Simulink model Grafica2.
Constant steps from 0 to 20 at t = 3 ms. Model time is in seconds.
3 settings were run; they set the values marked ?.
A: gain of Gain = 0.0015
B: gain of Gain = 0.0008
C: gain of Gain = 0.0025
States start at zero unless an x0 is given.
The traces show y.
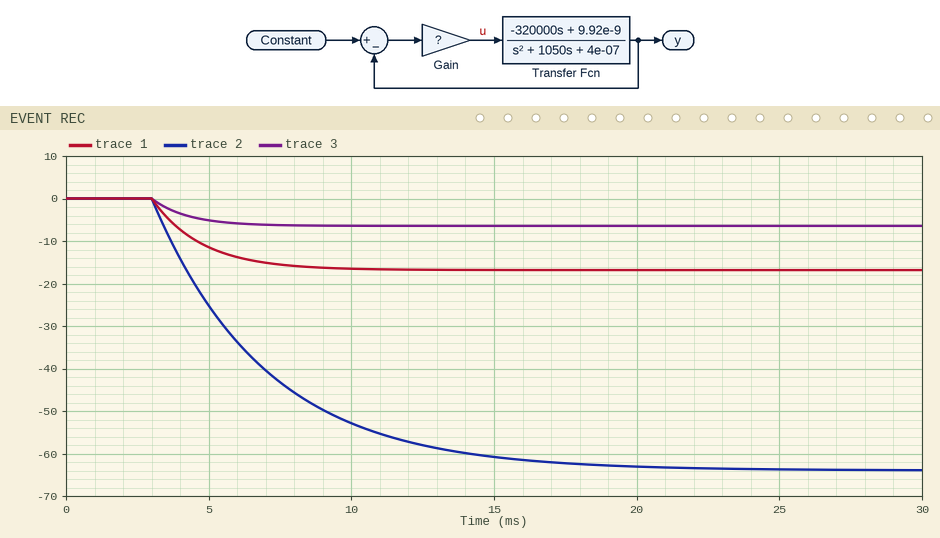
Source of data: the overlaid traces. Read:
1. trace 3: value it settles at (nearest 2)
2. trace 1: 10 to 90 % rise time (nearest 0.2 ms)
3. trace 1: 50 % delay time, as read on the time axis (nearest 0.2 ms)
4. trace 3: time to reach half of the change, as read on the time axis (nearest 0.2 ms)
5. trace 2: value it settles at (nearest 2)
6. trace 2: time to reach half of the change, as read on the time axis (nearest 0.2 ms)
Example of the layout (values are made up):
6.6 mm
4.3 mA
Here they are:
-6
3.8 ms
4.2 ms
3.8 ms
-64
5.8 ms
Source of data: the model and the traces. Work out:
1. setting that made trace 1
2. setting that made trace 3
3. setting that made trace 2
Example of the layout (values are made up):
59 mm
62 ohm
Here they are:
A
B
C
